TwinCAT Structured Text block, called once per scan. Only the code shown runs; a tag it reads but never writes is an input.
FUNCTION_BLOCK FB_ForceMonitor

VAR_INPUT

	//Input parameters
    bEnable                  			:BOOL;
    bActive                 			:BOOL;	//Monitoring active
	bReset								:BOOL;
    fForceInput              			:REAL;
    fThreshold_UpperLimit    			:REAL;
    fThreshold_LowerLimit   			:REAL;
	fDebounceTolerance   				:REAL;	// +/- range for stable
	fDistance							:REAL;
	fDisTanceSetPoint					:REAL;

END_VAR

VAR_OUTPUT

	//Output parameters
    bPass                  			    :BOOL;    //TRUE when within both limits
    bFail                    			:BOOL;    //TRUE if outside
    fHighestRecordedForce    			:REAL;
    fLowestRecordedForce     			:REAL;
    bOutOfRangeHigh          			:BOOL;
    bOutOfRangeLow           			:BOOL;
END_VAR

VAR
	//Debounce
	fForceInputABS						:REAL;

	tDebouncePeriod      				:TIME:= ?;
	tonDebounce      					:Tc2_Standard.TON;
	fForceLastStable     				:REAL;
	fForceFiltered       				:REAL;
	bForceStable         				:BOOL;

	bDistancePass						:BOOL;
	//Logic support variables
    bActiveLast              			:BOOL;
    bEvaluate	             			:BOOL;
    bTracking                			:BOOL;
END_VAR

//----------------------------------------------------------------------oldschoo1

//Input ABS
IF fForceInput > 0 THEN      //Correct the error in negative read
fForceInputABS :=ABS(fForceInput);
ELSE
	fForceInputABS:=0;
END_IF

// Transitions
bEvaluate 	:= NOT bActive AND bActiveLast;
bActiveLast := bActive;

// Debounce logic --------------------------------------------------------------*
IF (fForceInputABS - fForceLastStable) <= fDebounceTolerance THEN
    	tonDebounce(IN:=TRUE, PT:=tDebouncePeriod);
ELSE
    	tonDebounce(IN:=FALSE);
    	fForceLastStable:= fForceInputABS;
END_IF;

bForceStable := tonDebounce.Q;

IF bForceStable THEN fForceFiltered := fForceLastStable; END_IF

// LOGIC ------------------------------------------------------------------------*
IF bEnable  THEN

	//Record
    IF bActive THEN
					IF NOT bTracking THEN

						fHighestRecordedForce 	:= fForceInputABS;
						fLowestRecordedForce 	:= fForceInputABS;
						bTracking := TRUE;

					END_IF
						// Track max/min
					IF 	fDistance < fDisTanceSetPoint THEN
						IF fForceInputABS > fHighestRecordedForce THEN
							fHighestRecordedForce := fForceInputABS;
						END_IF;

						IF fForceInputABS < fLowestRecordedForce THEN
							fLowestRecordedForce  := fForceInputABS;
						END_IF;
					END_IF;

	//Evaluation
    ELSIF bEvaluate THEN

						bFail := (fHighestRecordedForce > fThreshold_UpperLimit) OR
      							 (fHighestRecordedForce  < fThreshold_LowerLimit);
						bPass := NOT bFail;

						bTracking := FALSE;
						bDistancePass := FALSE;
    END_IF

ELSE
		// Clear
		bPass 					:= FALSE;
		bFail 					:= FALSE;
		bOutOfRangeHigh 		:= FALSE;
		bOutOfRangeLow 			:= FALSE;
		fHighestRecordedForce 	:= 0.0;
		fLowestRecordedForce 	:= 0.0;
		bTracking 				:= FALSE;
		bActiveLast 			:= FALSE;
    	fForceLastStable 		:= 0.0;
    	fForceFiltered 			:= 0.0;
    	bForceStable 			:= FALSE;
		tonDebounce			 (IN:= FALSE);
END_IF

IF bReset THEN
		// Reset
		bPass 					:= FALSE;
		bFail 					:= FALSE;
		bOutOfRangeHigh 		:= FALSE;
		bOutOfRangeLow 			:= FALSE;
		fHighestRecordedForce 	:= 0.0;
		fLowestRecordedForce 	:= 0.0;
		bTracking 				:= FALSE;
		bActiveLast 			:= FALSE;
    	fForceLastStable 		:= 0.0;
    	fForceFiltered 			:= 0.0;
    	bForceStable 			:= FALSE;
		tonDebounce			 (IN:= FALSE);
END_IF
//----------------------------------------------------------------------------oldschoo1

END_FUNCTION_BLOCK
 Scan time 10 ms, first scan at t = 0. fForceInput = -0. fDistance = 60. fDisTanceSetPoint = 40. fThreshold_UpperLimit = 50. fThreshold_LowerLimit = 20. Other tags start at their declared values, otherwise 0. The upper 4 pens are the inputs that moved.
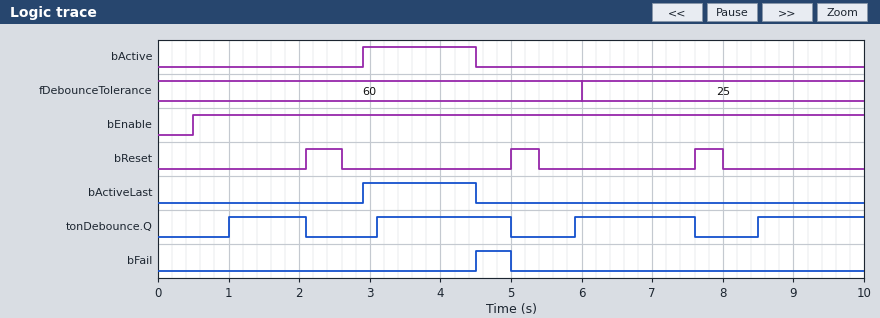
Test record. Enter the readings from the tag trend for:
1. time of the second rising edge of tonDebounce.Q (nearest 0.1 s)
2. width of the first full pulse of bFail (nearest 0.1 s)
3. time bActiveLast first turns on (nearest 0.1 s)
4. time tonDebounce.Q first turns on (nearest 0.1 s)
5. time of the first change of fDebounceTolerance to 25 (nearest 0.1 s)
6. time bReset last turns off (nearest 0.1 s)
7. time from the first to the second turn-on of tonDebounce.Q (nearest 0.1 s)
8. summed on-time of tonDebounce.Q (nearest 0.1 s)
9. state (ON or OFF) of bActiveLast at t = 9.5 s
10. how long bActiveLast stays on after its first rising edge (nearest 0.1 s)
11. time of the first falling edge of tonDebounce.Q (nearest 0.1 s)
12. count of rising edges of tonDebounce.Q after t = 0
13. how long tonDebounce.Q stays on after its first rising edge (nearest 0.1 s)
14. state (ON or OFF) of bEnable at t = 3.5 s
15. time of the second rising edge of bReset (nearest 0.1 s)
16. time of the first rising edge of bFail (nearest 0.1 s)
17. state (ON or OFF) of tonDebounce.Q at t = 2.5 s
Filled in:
3.1 s
0.5 s
2.9 s
1.0 s
6.0 s
8.0 s
2.1 s
6.2 s
OFF
1.6 s
2.1 s
4
1.1 s
ON
5.0 s
4.5 s
OFF
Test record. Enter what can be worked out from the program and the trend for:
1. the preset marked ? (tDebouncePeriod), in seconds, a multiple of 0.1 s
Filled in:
0.5 s
